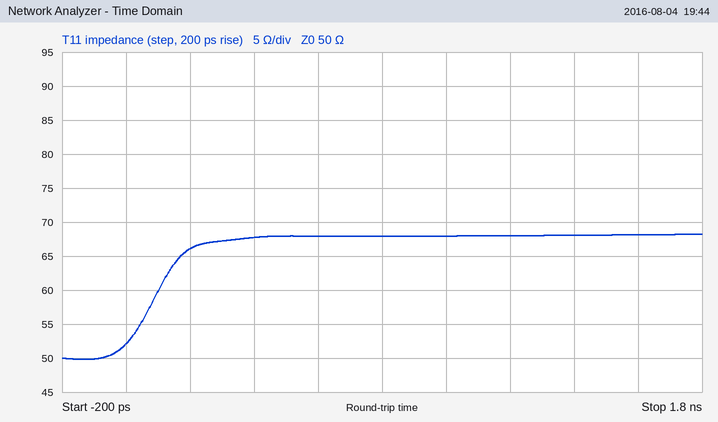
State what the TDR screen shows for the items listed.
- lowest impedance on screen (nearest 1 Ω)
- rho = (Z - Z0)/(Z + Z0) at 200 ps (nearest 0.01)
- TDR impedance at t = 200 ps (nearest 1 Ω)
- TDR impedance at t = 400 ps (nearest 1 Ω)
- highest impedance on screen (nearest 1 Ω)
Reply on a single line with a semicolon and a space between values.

50 Ω; +0.14; 66 Ω; 68 Ω; 68 Ω
